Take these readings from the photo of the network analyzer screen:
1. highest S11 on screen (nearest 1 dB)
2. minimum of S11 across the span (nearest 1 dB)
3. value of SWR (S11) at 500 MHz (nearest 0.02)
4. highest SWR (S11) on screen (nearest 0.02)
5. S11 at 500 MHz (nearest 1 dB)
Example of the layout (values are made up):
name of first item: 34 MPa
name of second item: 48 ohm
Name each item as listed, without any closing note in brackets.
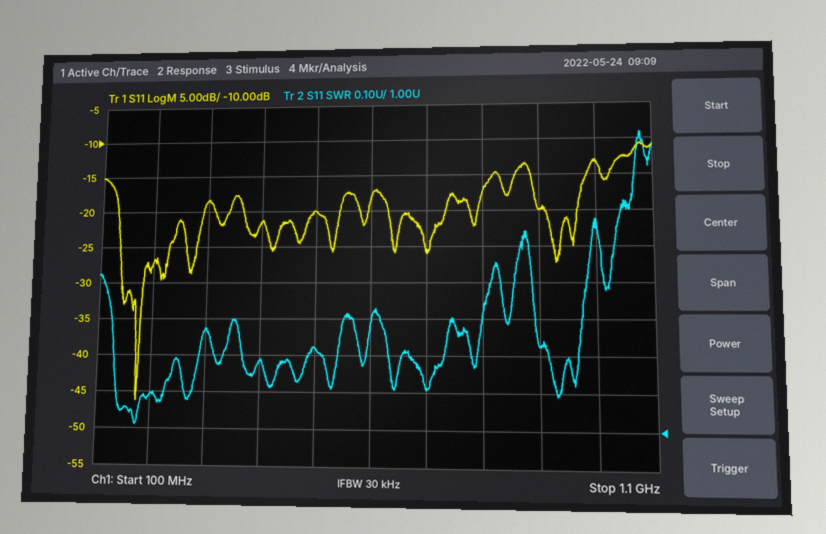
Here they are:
highest S11 on screen: -11 dB
minimum of S11 across the span: -46 dB
value of SWR (S11) at 500 MHz: 1.22
highest SWR (S11) on screen: 1.82
S11 at 500 MHz: -20 dB
